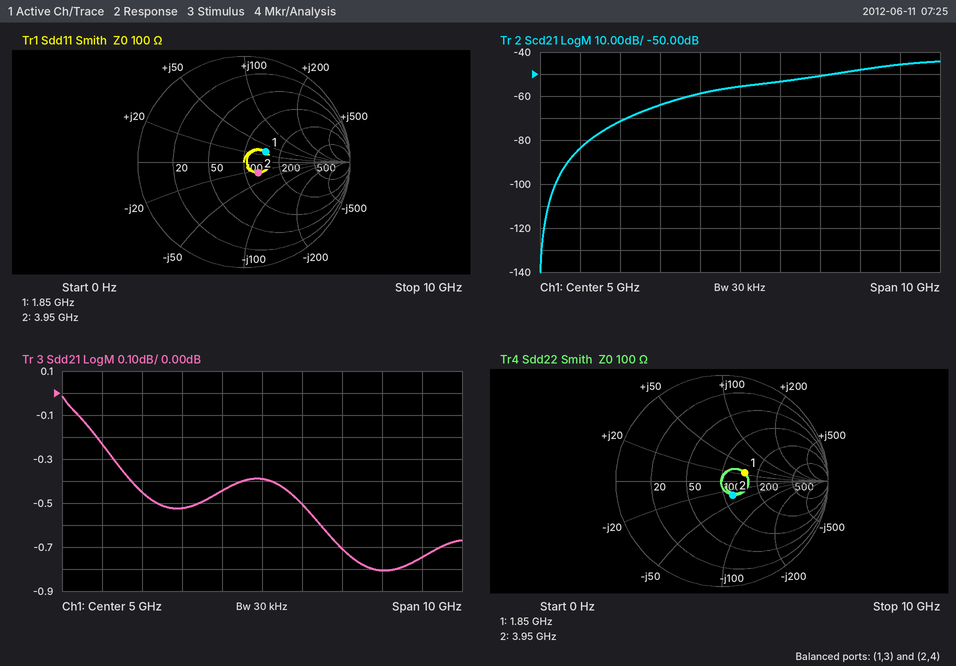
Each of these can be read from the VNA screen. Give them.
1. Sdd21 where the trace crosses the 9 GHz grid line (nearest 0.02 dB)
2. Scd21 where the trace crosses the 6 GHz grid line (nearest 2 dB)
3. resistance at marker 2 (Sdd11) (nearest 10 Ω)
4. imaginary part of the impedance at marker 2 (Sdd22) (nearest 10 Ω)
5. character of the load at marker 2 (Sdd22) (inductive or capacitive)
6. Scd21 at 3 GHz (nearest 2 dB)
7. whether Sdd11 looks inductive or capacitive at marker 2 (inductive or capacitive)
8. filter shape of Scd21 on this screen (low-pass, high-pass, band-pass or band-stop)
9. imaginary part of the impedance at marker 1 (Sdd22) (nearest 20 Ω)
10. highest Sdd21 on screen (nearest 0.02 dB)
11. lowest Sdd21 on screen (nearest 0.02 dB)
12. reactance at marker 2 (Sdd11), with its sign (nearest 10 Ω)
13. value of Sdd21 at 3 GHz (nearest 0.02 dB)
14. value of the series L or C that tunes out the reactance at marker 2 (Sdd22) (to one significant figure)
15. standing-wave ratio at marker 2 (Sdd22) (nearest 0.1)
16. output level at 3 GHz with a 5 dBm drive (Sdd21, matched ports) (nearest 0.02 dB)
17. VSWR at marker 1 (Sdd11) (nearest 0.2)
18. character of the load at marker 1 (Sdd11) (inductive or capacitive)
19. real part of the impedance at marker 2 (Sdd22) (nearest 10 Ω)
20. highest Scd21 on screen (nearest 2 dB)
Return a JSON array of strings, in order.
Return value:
["-0.74 dB", "-54 dB", "130 Ω", "-30 Ω", "capacitive", "-64 dB", "capacitive", "high-pass", "+20 Ω", "-0.02 dB", "-0.80 dB", "-30 Ω", "-0.52 dB", "1 nH", "1.4", "4.48 dBm", "1.6", "inductive", "120 Ω", "-44 dB"]
